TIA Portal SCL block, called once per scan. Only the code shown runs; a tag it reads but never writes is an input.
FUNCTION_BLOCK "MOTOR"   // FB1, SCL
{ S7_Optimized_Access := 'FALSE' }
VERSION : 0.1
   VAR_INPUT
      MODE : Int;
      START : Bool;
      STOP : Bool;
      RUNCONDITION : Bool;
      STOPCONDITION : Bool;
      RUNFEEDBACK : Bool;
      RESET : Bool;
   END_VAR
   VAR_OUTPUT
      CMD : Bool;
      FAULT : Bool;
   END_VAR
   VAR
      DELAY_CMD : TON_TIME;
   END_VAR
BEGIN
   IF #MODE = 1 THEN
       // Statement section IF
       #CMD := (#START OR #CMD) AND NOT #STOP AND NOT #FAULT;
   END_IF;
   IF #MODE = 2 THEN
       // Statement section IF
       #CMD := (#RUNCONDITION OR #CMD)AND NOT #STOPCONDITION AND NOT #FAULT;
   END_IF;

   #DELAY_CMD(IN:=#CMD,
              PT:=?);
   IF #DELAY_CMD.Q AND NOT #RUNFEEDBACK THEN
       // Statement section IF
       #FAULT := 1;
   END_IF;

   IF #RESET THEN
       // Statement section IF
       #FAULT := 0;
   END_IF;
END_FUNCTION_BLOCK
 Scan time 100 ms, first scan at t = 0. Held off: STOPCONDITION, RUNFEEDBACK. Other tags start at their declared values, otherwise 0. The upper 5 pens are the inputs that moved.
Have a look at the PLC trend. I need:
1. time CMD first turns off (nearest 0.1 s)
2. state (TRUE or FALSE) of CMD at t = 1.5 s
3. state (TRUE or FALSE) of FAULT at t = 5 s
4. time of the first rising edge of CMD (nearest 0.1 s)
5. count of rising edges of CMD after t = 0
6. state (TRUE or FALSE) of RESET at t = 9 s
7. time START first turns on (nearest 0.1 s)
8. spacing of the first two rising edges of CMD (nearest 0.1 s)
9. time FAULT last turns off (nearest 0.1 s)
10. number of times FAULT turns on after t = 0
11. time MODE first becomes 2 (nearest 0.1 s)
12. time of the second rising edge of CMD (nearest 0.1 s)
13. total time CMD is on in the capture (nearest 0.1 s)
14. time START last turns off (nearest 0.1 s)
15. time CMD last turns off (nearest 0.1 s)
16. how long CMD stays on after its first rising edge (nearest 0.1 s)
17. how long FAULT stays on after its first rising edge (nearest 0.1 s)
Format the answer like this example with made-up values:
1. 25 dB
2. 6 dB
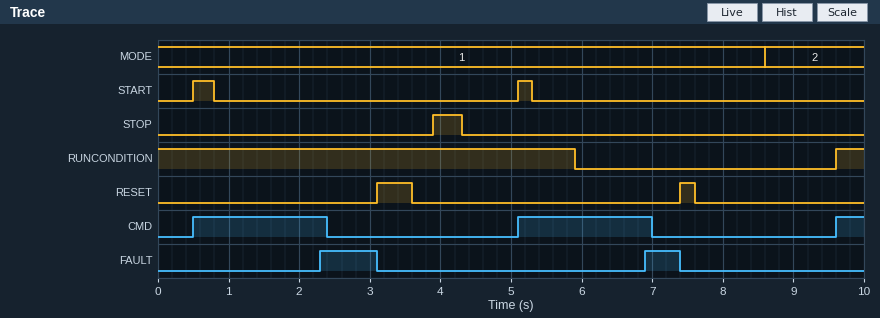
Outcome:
1. 2.4 s
2. TRUE
3. FALSE
4. 0.5 s
5. 3
6. FALSE
7. 0.5 s
8. 4.6 s
9. 7.4 s
10. 2
11. 8.6 s
12. 5.1 s
13. 4.2 s
14. 5.3 s
15. 7.0 s
16. 1.9 s
17. 0.8 s
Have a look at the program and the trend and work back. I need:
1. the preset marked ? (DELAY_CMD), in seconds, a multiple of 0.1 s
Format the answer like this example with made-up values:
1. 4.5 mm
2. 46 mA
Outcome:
1. 1.8 s
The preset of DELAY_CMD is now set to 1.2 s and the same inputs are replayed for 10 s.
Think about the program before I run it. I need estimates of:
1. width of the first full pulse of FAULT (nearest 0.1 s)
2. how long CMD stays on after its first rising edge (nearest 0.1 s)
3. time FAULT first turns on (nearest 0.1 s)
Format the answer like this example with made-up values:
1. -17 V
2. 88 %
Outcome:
1. 1.4 s
2. 1.3 s
3. 1.7 s
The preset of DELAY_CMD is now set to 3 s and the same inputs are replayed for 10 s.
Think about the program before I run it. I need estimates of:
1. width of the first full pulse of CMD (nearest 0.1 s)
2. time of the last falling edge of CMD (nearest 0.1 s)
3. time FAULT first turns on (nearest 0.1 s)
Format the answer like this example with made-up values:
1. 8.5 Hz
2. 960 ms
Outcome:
1. 3.2 s
2. 3.7 s
3. 3.6 s
